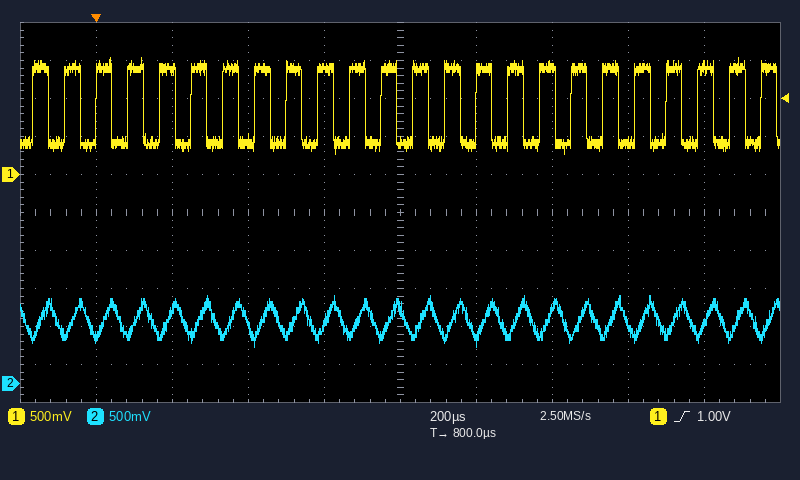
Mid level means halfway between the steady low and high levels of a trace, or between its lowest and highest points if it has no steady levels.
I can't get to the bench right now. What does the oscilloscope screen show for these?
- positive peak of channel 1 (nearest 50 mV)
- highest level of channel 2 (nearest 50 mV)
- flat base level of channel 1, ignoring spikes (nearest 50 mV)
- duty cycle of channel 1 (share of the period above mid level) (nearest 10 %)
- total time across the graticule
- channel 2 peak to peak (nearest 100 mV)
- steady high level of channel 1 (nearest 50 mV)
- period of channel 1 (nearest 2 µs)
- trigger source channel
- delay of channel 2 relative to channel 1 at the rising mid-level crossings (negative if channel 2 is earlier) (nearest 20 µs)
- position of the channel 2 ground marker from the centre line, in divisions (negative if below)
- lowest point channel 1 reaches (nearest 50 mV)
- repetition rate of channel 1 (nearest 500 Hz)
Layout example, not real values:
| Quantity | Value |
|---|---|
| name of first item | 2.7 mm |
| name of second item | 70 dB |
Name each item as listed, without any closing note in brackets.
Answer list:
| Quantity | Value |
|---|---|
| positive peak of channel 1 | 1.55 V |
| highest level of channel 2 | 1.15 V |
| flat base level of channel 1, ignoring spikes | 400 mV |
| duty cycle of channel 1 (share of the period above mid level) | 50 % |
| total time across the graticule | 2 ms |
| channel 2 peak to peak | 700 mV |
| steady high level of channel 1 | 1.40 V |
| period of channel 1 | 84 µs |
| trigger source channel | channel 1 |
| delay of channel 2 relative to channel 1 at the rising mid-level crossings (negative if channel 2 is earlier) | +20 µs |
| position of the channel 2 ground marker from the centre line, in divisions | -4.5 div |
| lowest point channel 1 reaches | 250 mV |
| repetition rate of channel 1 | 12.0 kHz |
